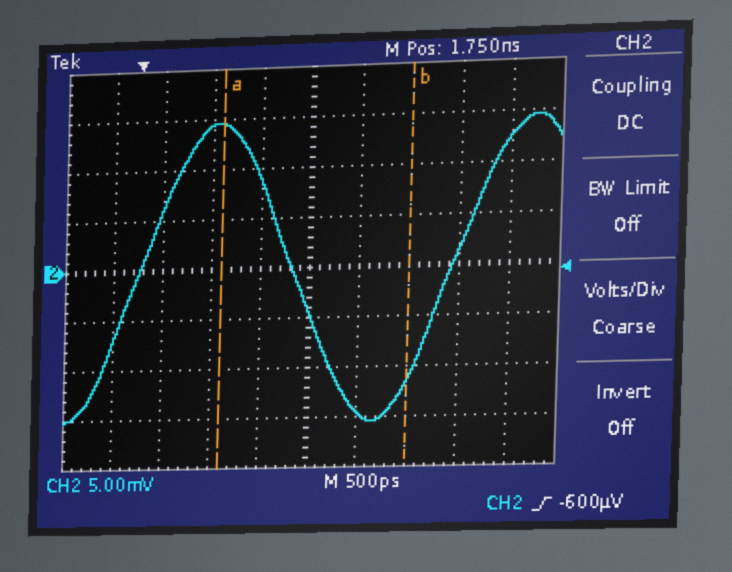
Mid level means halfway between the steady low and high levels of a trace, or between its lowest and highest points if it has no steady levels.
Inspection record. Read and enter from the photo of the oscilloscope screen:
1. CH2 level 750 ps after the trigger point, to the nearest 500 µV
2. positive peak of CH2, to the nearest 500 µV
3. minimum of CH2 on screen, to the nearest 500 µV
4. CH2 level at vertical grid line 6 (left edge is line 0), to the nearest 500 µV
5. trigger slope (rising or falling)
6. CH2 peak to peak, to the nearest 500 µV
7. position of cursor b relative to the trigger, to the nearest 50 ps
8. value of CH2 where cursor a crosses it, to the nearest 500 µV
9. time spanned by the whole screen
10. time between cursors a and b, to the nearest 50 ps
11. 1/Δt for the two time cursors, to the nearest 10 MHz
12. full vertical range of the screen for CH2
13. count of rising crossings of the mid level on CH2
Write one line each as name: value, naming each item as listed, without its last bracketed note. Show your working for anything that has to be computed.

CH2 level 750 ps after the trigger point, to the nearest 500 µV: 14.5 mV
positive peak of CH2, to the nearest 500 µV: 14.5 mV
minimum of CH2 on screen, to the nearest 500 µV: -15.5 mV
CH2 level at vertical grid line 6 (left edge is line 0), to the nearest 500 µV: -14.5 mV
trigger slope: rising
CH2 peak to peak, to the nearest 500 µV: 14.5 mV − (-15.5 mV) = 30.0 mV
position of cursor b relative to the trigger, to the nearest 50 ps: +2.75 ns
value of CH2 where cursor a crosses it, to the nearest 500 µV: 14.5 mV
time spanned by the whole screen: 5 ns
time between cursors a and b, to the nearest 50 ps: 1.90 ns
1/Δt for the two time cursors, to the nearest 10 MHz: 1 / 1.90 ns ≈ 530 MHz
full vertical range of the screen for CH2: 40 mV
count of rising crossings of the mid level on CH2: 2
